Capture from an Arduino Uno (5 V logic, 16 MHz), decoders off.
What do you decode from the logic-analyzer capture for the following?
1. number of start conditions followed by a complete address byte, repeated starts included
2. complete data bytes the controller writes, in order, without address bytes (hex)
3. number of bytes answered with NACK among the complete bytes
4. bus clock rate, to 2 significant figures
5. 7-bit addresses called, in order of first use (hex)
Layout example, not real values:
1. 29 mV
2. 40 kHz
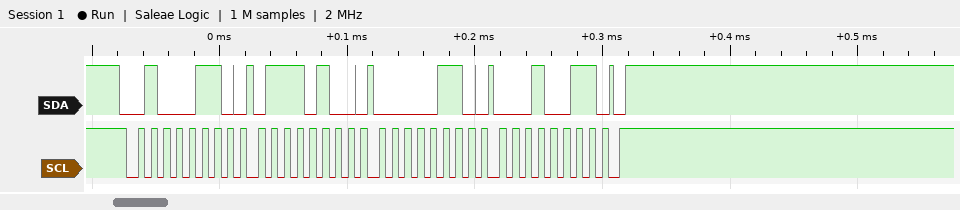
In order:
1. 1
2. 74 06 13
3. 0
4. 100 kHz
5. 0x23
